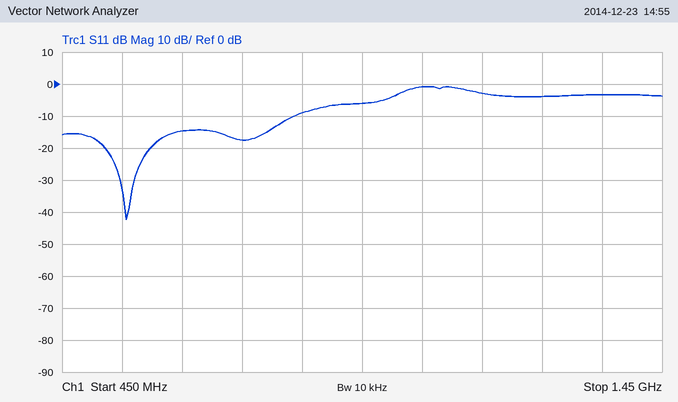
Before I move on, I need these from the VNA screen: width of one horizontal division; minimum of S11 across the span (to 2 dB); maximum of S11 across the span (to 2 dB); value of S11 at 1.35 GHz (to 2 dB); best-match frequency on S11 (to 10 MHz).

100 MHz
-42 dB
0 dB
-4 dB
560 MHz
